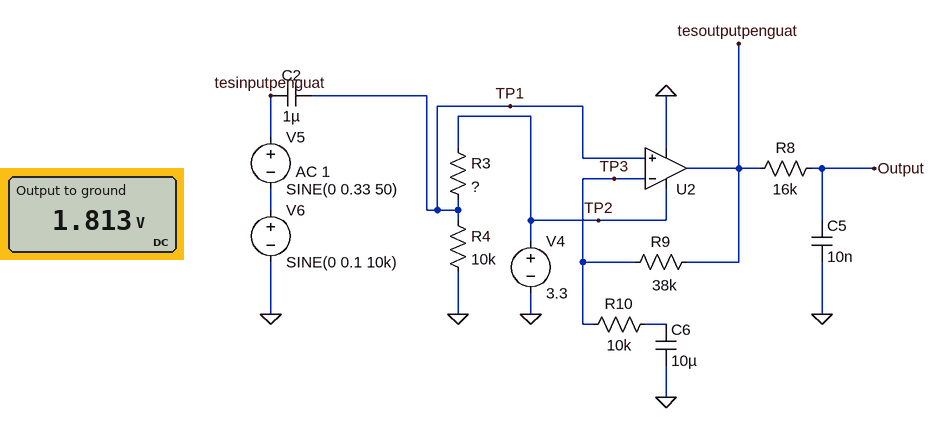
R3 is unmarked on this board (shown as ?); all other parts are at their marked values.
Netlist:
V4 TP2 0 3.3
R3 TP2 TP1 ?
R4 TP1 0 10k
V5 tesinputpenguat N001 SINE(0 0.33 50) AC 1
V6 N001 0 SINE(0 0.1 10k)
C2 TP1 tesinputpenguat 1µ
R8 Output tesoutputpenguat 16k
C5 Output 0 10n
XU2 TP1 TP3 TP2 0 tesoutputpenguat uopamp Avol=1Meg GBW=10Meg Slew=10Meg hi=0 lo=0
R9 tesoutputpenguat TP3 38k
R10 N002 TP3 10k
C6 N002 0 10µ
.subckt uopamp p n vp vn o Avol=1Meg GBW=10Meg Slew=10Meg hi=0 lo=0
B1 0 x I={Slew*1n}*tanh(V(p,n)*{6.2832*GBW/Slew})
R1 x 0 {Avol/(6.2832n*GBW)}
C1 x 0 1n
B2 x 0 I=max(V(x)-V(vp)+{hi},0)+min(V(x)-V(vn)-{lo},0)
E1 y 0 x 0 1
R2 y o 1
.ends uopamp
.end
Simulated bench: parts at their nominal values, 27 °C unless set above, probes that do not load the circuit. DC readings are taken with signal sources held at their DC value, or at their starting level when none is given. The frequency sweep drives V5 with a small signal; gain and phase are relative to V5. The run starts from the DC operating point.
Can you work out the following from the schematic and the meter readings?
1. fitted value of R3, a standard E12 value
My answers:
8.2 kΩ
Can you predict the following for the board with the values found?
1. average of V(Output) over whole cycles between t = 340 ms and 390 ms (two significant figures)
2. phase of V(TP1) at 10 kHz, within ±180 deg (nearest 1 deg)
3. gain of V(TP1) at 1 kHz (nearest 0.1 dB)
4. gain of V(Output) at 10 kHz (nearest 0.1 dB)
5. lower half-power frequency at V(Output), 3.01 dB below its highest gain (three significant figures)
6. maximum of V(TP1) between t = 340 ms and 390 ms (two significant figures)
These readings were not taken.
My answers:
1.8 V
0 deg
0 dB
-6.5 dB
33.1 Hz
2.2 V
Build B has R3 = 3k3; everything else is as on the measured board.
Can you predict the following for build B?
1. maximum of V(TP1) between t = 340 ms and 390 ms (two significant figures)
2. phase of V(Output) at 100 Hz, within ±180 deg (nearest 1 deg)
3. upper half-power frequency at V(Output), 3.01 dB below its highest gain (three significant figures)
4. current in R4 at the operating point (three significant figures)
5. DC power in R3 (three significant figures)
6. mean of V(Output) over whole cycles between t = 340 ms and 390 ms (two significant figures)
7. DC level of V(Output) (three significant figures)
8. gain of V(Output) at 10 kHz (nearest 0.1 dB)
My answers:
2.8 V
28 deg
1.12 kHz
248 µA
203 µW
2.5 V
2.48 V
-6.5 dB
